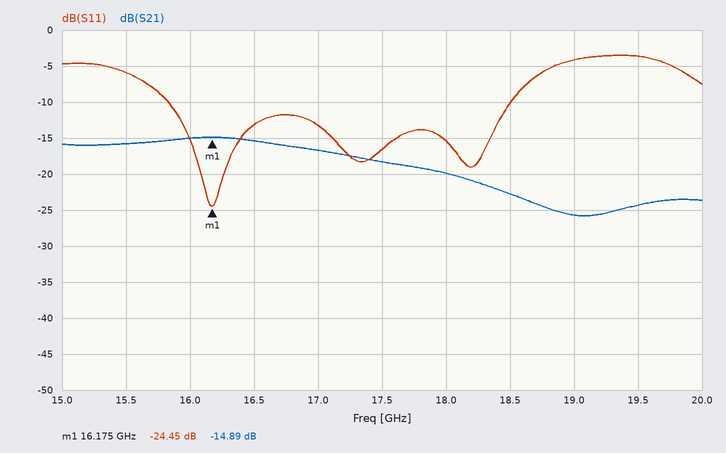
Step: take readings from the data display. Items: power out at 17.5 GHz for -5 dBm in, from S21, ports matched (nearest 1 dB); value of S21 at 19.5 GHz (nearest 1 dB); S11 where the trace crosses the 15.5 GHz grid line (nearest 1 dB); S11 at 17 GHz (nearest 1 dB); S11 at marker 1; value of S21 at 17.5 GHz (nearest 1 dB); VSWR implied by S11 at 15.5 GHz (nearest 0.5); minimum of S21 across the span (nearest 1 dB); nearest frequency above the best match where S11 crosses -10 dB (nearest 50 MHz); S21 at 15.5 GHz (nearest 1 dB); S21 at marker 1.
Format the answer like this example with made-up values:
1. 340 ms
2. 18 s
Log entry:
1. -23 dBm
2. -24 dB
3. -6 dB
4. -13 dB
5. -24.45 dB
6. -18 dB
7. 3.0
8. -26 dB
9. 18.50 GHz
10. -16 dB
11. -14.89 dB
